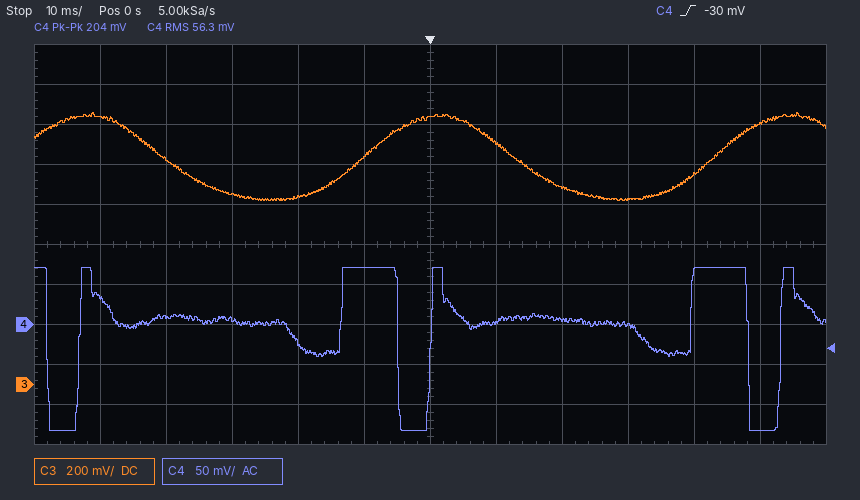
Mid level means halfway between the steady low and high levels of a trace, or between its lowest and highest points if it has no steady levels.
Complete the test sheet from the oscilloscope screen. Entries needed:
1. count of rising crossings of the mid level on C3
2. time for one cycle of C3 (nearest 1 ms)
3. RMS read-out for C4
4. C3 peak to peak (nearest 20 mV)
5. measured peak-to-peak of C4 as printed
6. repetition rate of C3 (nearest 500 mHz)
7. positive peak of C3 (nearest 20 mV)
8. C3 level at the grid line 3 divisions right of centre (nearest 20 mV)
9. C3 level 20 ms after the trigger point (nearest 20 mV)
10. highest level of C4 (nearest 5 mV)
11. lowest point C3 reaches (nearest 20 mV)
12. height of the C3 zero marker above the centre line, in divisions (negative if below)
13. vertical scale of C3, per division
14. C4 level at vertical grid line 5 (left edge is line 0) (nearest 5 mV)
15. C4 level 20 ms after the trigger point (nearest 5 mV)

2
53 ms
56.3 mV
440 mV
204 mV
19.0 Hz
1.36 V
920 mV
980 mV
70 mV
920 mV
-3.5 div
200 mV
70 mV
5 mV
